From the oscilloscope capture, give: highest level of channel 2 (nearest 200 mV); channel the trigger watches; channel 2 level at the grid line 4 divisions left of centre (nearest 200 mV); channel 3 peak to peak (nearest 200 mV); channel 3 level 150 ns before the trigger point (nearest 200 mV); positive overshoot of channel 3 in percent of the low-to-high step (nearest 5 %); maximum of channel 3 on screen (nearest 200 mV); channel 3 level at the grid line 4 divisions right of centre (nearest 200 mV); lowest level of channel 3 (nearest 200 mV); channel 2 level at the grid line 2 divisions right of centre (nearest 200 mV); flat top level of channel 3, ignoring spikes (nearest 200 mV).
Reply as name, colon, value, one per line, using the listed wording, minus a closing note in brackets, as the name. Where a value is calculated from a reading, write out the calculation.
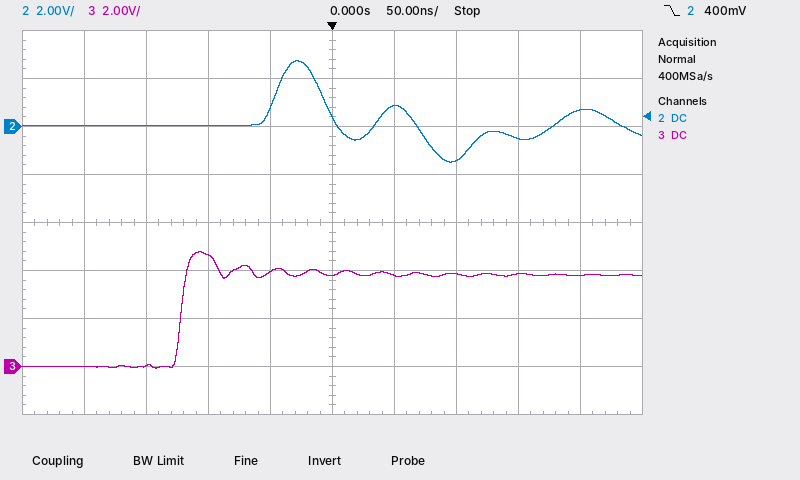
highest level of channel 2: 2.8 V
channel the trigger watches: channel 2
channel 2 level at the grid line 4 divisions left of centre: 0.0 V
channel 3 peak to peak: 4.8 V − (0.0 V) = 4.8 V
channel 3 level 150 ns before the trigger point: 0.0 V
positive overshoot of channel 3 in percent of the low-to-high step: 25 %
maximum of channel 3 on screen: 4.8 V
channel 3 level at the grid line 4 divisions right of centre: 3.8 V
lowest level of channel 3: 0.0 V
channel 2 level at the grid line 2 divisions right of centre: -1.4 V
flat top level of channel 3, ignoring spikes: 3.8 V
